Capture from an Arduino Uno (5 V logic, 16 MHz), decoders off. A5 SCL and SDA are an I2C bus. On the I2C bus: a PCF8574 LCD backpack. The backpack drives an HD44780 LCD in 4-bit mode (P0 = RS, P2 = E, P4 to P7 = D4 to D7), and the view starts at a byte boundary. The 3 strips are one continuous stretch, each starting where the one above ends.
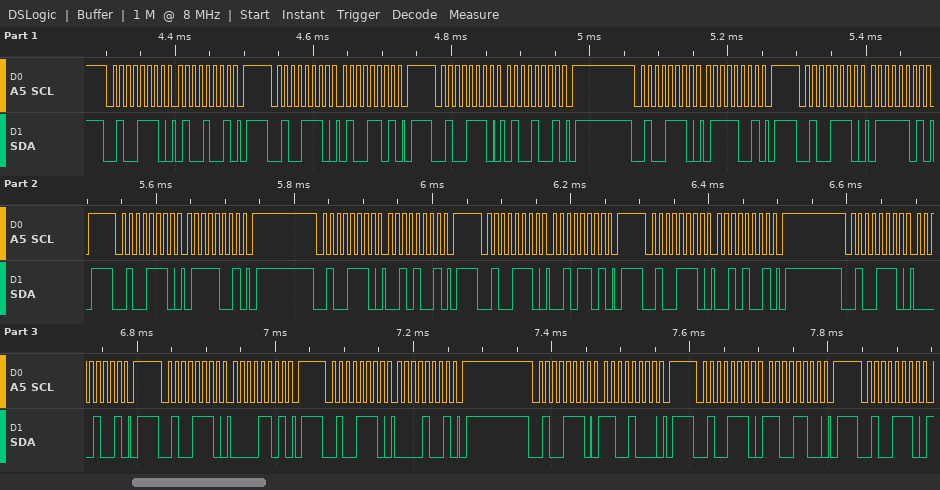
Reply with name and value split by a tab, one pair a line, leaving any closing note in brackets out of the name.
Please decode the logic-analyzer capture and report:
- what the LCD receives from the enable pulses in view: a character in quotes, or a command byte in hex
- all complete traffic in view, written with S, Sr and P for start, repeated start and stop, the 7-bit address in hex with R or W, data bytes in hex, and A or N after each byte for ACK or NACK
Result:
what the LCD receives from the enable pulses in view: a character in quotes, or a command byte in hex	'G' ' '
all complete traffic in view, written with S, Sr and P for start, repeated start and stop, the 7-bit address in hex with R or W, data bytes in hex, and A or N after each byte for ACK or NACK	S 27W A 49 A P S 27W A 4D A P S 27W A 49 A P S 27W A 79 A P S 27W A 7D A P S 27W A 79 A P S 27W A 29 A P S 27W A 2D A P S 27W A 29 A P S 27W A 09 A P S 27W A 0D A P S 27W A 09 A P S 27W A C8 A P S 27W A CC A P S 27W A
